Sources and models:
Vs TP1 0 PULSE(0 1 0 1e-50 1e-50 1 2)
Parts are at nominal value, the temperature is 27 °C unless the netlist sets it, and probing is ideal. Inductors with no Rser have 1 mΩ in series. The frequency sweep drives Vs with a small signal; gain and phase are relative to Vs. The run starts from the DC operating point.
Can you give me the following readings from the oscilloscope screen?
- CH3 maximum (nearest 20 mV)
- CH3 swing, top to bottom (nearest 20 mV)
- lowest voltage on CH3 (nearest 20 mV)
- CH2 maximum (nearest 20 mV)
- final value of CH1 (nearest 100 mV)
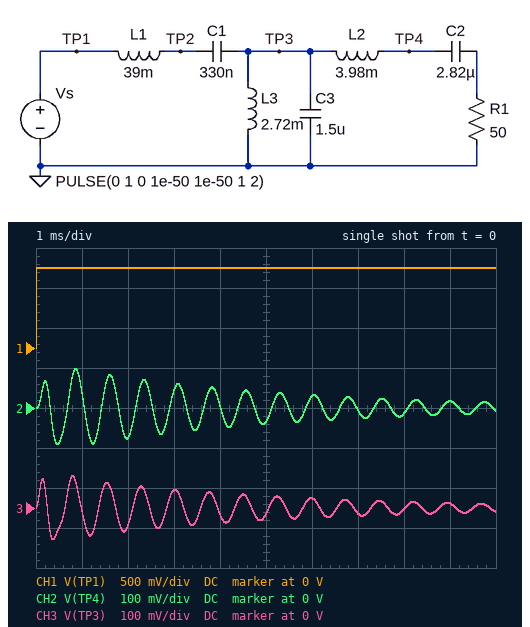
80 mV
160 mV
-80 mV
100 mV
1.0 V
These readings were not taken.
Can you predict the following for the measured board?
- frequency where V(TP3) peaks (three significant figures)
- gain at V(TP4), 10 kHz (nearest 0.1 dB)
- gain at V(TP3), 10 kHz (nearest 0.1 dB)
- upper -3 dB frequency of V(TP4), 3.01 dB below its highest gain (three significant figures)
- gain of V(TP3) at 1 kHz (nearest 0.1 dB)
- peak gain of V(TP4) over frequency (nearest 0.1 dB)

1.35 kHz
-60.0 dB
-46.1 dB
1.39 kHz
-19.2 dB
6.9 dB
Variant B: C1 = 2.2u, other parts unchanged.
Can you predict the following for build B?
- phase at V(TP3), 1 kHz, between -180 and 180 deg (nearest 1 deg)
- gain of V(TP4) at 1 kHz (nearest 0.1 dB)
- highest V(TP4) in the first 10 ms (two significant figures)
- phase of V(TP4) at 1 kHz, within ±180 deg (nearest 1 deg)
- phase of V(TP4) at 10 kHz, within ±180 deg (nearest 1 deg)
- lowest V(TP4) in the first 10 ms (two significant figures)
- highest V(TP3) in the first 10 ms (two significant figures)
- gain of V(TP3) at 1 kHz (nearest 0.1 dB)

-17 deg
-16.3 dB
94 mV
-34 deg
96 deg
-84 mV
91 mV
-18.4 dB
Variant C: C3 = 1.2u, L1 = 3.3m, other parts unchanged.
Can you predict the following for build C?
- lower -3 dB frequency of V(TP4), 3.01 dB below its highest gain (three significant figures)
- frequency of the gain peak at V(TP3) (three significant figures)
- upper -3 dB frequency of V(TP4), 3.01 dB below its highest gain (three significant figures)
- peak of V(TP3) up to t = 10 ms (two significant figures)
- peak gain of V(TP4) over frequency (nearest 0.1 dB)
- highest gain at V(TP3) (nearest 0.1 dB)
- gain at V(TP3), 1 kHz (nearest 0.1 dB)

5.72 kHz
5.79 kHz
5.86 kHz
290 mV
12.0 dB
21.0 dB
-25.8 dB
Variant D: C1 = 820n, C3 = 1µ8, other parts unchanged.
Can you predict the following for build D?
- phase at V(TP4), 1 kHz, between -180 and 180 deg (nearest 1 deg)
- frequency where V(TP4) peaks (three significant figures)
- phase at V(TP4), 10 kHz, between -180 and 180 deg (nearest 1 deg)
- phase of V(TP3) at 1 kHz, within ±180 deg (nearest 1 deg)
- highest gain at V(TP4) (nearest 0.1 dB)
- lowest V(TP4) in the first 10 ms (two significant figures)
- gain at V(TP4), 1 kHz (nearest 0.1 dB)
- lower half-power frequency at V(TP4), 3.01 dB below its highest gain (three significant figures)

-30 deg
851 Hz
96 deg
-14 deg
15.0 dB
-100 mV
-7.5 dB
843 Hz
